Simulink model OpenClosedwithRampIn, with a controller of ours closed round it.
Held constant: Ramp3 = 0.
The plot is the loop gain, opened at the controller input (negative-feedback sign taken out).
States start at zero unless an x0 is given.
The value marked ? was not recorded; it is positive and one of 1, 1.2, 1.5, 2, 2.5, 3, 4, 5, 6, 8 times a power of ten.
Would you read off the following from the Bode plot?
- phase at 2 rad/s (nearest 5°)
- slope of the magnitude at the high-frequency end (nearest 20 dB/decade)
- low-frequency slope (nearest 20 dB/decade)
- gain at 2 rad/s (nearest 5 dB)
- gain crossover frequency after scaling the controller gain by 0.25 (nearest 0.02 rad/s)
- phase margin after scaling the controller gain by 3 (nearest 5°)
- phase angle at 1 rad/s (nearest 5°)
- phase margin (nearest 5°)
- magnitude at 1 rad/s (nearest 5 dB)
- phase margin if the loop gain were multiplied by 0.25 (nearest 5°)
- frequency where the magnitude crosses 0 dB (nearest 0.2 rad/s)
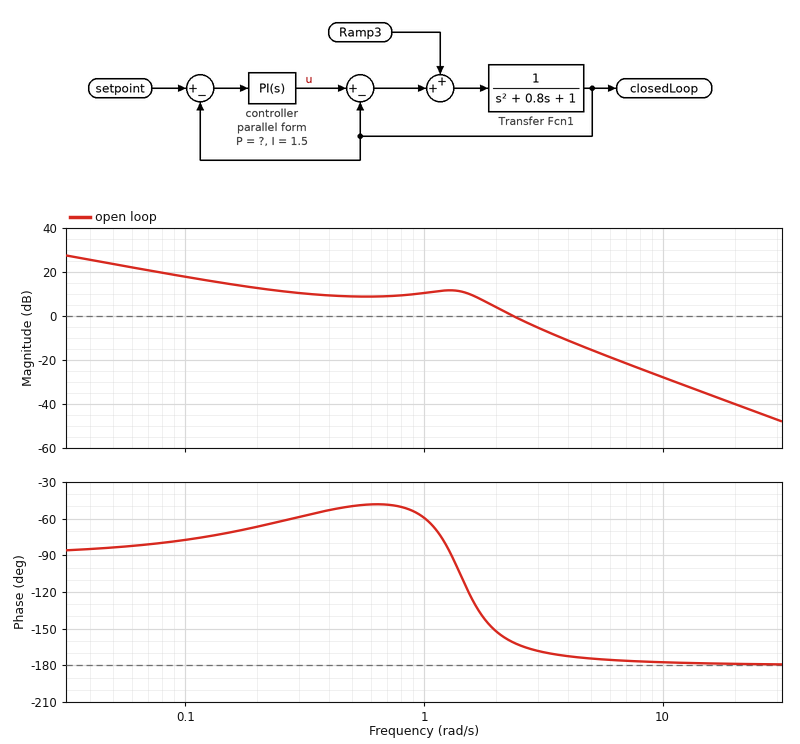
-150°
-40 dB/decade
-20 dB/decade
5 dB
0.22 rad/s
10°
-60°
20°
10 dB
115°
2.4 rad/s
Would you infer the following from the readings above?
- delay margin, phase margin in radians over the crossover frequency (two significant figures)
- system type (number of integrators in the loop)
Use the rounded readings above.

0.15 s
1
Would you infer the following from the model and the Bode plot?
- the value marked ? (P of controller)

4
